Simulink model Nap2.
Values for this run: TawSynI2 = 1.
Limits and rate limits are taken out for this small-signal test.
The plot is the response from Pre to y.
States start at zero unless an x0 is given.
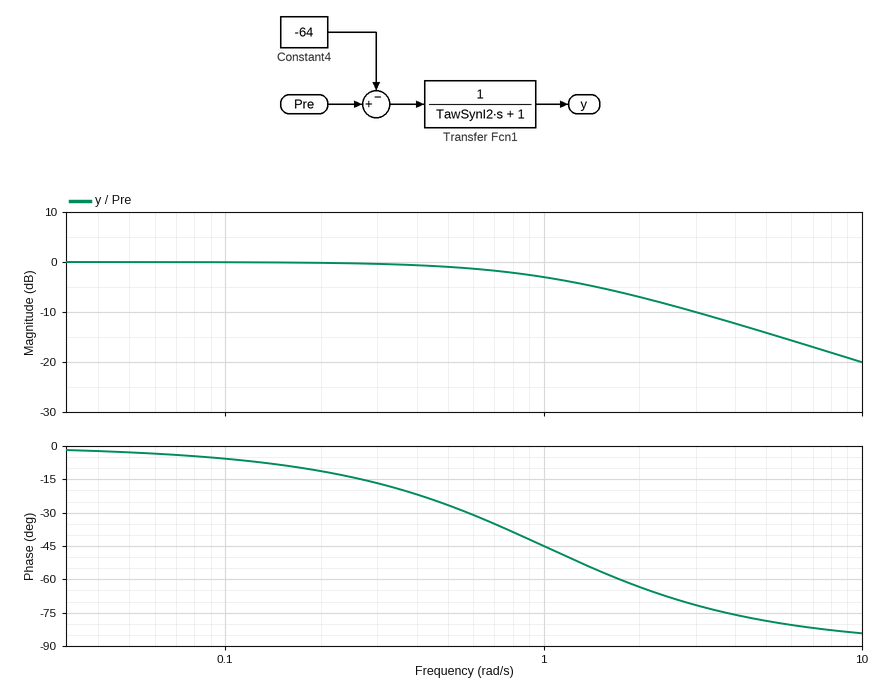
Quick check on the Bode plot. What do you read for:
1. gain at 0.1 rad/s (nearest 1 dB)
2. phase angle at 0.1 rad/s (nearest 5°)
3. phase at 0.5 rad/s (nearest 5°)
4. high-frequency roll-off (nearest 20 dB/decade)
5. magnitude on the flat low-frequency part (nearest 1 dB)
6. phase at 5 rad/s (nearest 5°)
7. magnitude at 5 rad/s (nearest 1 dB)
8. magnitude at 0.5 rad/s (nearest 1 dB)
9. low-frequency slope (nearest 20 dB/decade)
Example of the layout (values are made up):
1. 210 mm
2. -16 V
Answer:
1. 0 dB
2. -5°
3. -25°
4. -20 dB/decade
5. 0 dB
6. -80°
7. -14 dB
8. -1 dB
9. 0 dB/decade
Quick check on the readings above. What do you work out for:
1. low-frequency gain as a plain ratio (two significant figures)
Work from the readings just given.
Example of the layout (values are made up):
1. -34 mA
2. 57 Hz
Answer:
1. 1.0
